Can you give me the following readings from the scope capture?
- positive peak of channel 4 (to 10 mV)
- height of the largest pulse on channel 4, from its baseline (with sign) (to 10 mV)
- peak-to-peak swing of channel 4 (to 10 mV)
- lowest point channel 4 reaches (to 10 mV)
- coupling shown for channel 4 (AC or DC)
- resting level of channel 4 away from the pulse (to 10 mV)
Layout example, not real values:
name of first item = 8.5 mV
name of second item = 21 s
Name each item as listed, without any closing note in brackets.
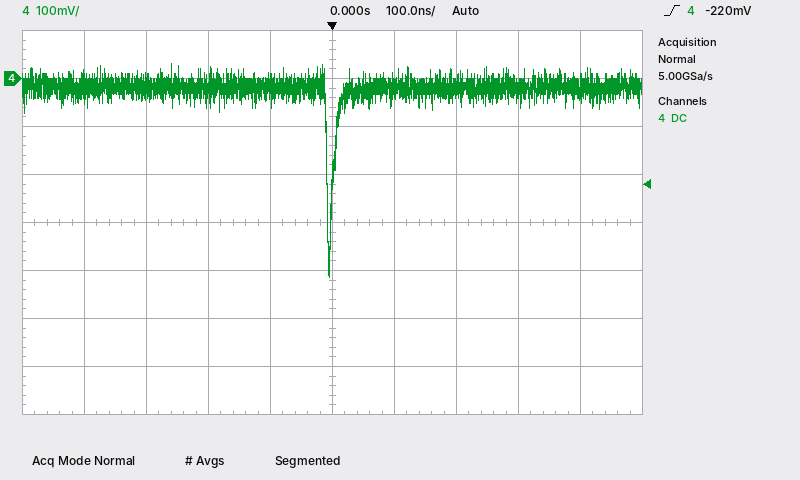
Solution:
positive peak of channel 4 = 30 mV
height of the largest pulse on channel 4, from its baseline (with sign) = -390 mV
peak-to-peak swing of channel 4 = 440 mV
lowest point channel 4 reaches = -410 mV
coupling shown for channel 4 = DC
resting level of channel 4 away from the pulse = -20 mV
